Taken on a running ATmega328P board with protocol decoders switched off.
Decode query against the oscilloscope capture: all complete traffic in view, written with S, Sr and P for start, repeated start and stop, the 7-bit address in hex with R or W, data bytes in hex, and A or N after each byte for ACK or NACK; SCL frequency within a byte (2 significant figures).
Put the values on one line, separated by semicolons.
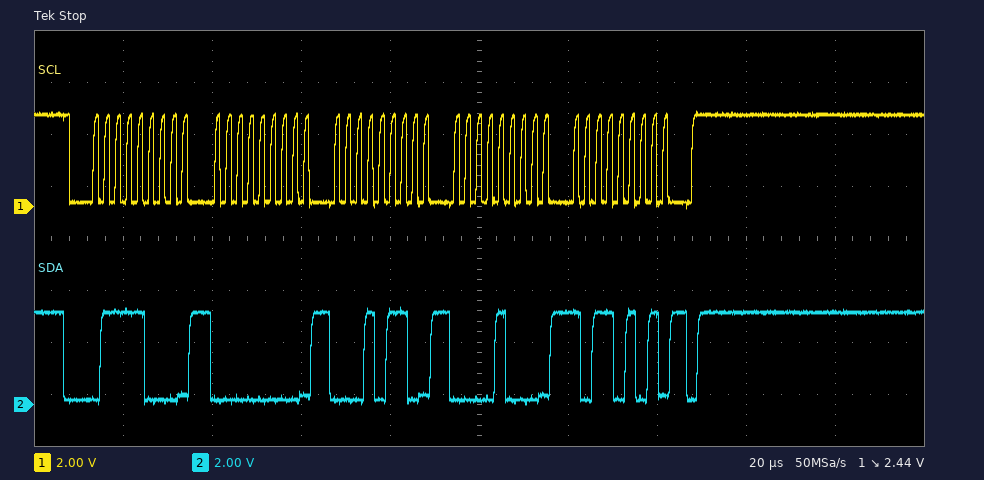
S 3CW A 00 A 16 A 08 A B5 A P; 400 kHz
